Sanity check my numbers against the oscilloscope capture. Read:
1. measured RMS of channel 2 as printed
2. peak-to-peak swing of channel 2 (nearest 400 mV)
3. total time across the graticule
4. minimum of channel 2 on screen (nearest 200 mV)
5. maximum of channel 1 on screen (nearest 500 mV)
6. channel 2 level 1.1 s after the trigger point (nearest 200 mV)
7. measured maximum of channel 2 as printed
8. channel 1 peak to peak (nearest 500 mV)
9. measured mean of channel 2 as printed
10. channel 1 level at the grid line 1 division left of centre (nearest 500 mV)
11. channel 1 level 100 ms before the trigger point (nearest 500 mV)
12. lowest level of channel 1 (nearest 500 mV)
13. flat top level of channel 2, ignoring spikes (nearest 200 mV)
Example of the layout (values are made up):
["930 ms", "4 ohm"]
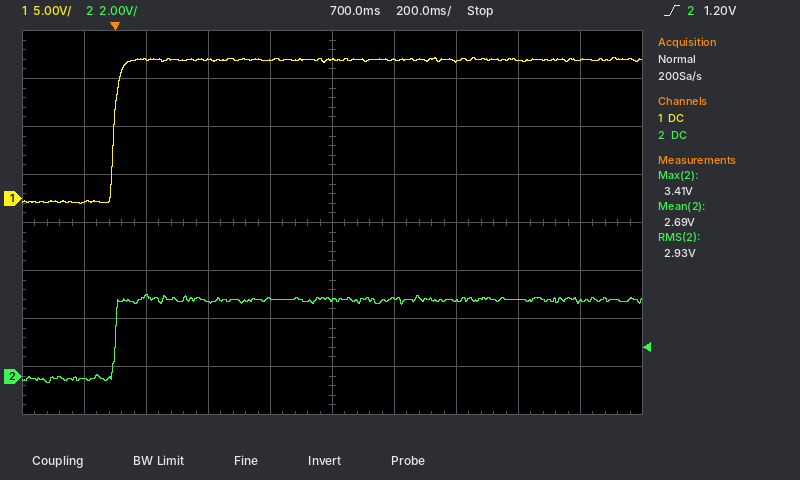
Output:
["2.93 V", "3.6 V", "2 s", "-200 mV", "14.5 V", "3.2 V", "3.41 V", "15.0 V", "2.69 V", "14.5 V", "-500 mV", "-500 mV", "3.2 V"]
